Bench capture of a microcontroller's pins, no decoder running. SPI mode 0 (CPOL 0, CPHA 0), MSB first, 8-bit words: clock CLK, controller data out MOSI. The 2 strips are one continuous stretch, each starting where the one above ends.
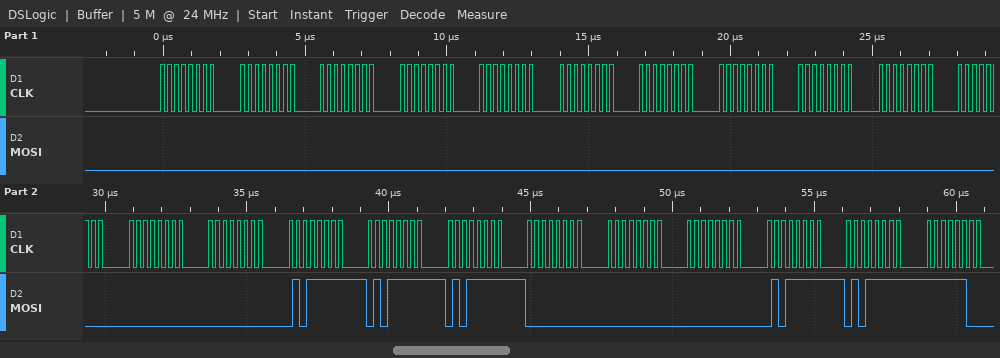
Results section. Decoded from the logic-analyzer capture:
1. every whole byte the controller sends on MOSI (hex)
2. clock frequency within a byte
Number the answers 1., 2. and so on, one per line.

1. 00 00 00 00 00 00 00 00 00 00 00 00 00 5F 5F 5F 00 00 00 5F 5F FC
2. 4 MHz
